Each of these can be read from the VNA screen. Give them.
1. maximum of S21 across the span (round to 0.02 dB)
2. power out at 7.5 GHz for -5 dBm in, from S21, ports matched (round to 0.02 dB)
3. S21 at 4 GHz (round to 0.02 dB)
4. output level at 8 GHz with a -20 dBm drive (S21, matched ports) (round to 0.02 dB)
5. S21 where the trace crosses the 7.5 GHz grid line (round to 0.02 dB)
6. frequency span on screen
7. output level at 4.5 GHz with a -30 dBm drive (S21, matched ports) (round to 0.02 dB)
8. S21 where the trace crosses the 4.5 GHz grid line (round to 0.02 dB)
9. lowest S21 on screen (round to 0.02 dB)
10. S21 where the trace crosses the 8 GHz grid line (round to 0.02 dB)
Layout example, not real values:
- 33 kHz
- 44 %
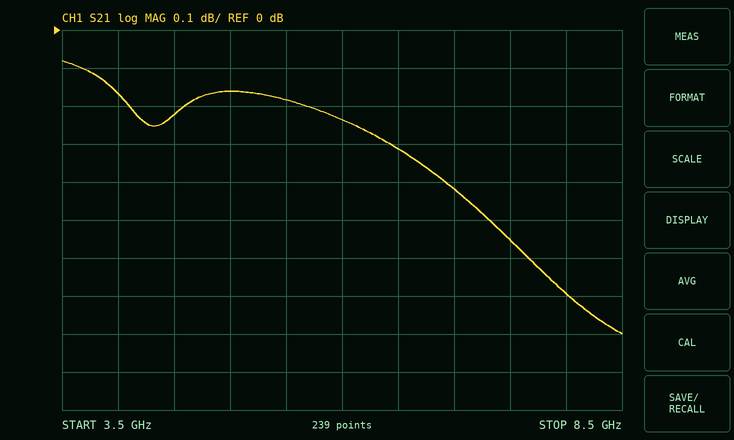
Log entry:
- -0.08 dB
- -5.56 dBm
- -0.16 dB
- -20.70 dBm
- -0.56 dB
- 5 GHz
- -30.22 dBm
- -0.22 dB
- -0.80 dB
- -0.70 dB
